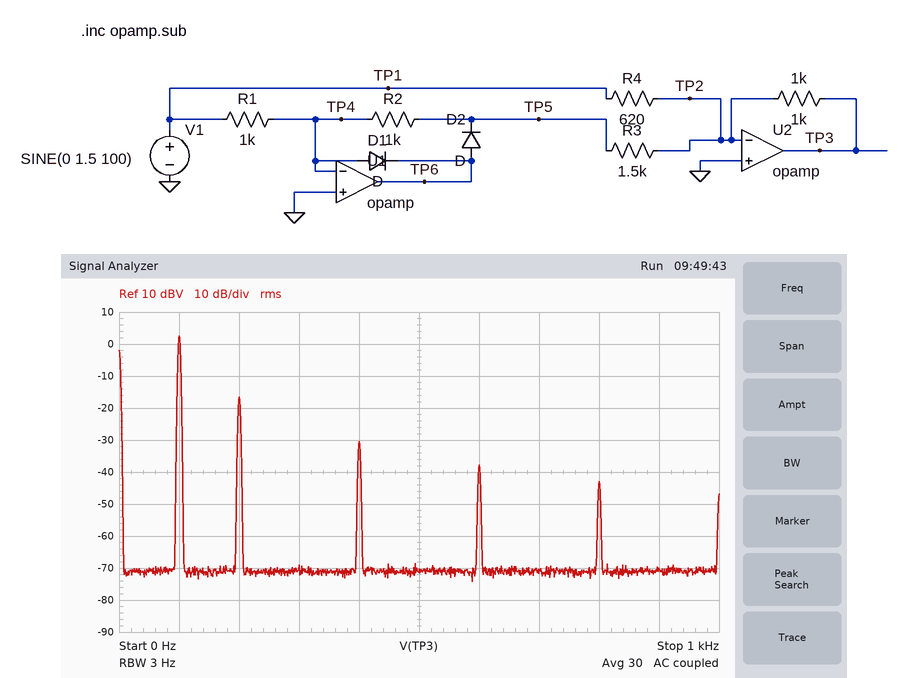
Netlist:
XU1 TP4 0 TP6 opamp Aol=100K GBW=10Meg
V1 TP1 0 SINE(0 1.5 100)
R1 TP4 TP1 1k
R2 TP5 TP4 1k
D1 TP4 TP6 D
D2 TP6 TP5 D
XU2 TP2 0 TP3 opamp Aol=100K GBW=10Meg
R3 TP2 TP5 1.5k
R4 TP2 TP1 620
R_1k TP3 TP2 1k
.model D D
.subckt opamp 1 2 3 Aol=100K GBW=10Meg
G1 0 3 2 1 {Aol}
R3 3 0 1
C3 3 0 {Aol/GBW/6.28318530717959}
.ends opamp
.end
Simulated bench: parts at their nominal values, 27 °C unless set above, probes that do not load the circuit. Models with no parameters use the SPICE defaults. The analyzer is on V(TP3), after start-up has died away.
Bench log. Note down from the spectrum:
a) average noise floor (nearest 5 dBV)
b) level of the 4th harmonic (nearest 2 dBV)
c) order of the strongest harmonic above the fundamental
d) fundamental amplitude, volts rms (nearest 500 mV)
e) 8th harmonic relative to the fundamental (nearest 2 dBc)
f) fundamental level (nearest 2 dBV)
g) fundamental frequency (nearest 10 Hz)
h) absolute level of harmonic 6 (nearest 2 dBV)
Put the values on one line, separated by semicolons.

-70 dBV; -30 dBV; 2; 1.5 V; -46 dBc; 2 dBV; 100 Hz; -38 dBV
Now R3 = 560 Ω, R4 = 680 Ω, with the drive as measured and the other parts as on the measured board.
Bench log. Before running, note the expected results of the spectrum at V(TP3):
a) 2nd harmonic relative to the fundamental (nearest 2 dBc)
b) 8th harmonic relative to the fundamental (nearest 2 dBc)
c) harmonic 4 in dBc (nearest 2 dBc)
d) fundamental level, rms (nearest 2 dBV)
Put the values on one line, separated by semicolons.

-4 dBc; -30 dBc; -18 dBc; -4 dBV
